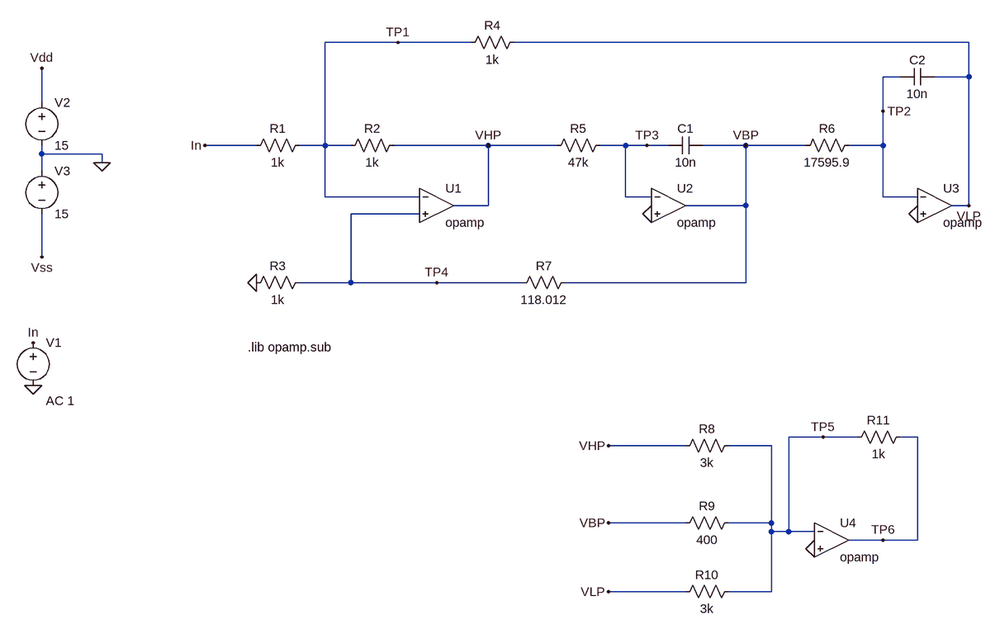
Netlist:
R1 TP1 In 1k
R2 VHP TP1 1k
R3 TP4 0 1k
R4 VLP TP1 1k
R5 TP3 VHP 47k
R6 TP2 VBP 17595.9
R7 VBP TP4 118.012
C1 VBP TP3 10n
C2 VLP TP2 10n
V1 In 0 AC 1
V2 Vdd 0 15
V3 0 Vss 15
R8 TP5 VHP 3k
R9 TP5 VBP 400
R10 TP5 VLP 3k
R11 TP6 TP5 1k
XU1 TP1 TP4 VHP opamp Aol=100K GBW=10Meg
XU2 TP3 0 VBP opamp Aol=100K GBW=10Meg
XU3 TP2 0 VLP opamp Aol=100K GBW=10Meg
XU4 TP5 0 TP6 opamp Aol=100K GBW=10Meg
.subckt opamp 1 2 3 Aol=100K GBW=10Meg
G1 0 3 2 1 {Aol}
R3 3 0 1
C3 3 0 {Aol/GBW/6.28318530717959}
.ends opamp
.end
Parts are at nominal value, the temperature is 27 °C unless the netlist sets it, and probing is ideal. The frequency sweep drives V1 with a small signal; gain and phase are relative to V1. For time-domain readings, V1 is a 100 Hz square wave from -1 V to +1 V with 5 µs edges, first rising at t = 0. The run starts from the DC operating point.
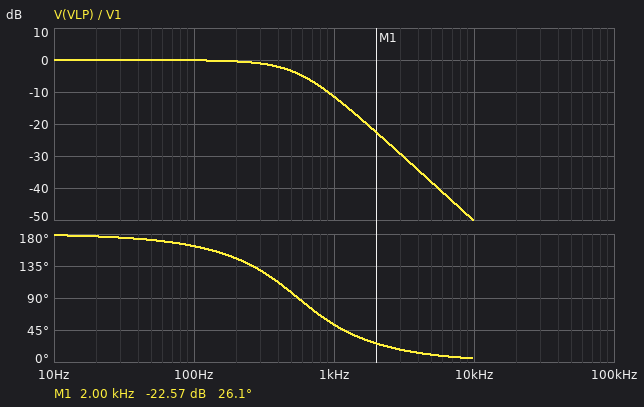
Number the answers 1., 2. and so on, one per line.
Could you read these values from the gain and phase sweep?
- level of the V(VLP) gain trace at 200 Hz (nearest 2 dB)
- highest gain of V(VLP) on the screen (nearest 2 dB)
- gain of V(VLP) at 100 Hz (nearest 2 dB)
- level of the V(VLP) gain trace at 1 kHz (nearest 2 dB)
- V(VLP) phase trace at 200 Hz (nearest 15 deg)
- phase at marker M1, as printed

1. 0 dB
2. 0 dB
3. 0 dB
4. -12 dB
5. 150 deg
6. 26.1 deg
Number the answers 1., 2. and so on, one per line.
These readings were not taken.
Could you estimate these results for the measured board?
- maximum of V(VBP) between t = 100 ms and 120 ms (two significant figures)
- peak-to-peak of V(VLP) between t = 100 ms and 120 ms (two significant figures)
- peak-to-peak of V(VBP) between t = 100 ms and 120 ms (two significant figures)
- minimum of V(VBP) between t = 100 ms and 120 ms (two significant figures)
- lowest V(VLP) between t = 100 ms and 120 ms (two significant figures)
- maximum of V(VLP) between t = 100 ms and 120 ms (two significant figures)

1. 510 mV
2. 2.0 V
3. 1.0 V
4. -510 mV
5. -1.0 V
6. 1.0 V
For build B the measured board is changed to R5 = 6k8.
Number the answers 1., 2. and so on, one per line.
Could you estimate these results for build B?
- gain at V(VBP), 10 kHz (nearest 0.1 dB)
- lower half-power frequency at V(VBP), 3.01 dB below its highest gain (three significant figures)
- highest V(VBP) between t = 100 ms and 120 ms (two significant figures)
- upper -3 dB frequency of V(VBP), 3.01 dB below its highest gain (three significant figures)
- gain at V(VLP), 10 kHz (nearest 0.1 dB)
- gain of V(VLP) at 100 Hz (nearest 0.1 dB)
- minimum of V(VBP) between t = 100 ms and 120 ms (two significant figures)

1. -13.9 dB
2. 321 Hz
3. 660 mV
4. 6.61 kHz
5. -34.8 dB
6. -0.3 dB
7. -660 mV
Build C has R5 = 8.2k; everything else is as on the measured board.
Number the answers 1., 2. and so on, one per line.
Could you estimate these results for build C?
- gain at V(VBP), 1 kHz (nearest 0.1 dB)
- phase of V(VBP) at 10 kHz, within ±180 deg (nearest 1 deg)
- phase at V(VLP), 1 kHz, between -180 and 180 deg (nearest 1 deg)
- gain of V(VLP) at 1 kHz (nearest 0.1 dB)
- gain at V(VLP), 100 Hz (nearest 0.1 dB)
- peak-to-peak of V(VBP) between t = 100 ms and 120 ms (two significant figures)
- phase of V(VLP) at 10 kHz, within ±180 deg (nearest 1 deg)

1. -8.7 dB
2. -62 deg
3. 98 deg
4. -9.5 dB
5. -0.3 dB
6. 1.3 V
7. 28 deg
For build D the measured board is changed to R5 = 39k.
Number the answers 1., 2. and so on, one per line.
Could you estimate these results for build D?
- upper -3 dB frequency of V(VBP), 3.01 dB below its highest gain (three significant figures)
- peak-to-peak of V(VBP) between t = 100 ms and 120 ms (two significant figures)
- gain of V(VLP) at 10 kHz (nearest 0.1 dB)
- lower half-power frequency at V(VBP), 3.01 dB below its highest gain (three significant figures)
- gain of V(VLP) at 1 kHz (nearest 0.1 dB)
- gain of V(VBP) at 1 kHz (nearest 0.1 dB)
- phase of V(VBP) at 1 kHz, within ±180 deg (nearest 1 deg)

1. 1.37 kHz
2. 1.1 V
3. -48.7 dB
4. 270 Hz
5. -10.7 dB
6. -9.8 dB
7. -30 deg
